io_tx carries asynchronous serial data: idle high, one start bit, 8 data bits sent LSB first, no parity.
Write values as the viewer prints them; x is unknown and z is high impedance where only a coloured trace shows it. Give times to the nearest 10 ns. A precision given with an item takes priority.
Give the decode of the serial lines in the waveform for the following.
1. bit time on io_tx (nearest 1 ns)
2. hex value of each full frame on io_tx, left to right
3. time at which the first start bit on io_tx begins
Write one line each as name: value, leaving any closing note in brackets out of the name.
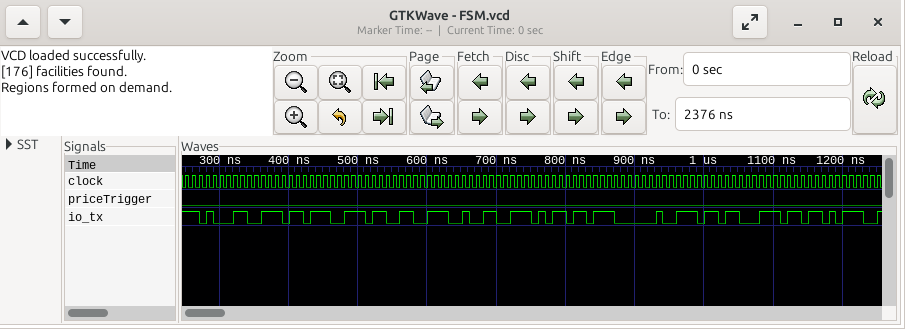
bit time on io_tx: 10 ns
hex value of each full frame on io_tx, left to right: 31, 3B, 33, 32, 6D, 20, 1B, 5B
time at which the first start bit on io_tx begins: 270 ns
